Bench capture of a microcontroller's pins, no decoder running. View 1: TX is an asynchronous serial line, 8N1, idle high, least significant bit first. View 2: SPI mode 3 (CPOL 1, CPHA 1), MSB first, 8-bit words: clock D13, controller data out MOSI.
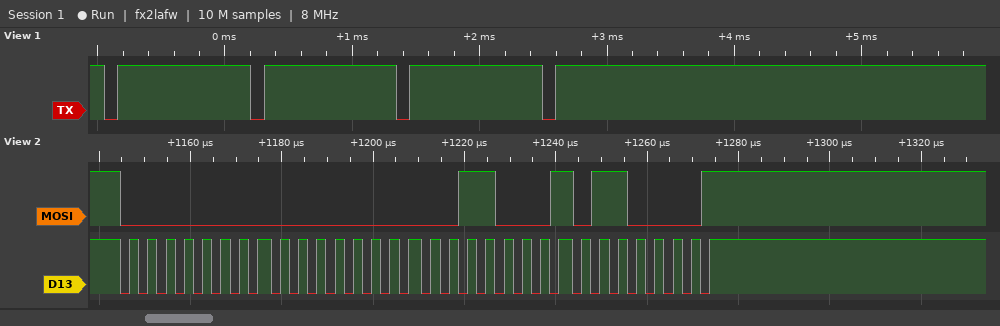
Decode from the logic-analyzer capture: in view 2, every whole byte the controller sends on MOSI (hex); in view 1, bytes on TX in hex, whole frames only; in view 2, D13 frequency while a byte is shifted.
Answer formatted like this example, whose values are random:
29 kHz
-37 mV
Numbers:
00 00 31 61
FF FF FF FF
250 kHz
